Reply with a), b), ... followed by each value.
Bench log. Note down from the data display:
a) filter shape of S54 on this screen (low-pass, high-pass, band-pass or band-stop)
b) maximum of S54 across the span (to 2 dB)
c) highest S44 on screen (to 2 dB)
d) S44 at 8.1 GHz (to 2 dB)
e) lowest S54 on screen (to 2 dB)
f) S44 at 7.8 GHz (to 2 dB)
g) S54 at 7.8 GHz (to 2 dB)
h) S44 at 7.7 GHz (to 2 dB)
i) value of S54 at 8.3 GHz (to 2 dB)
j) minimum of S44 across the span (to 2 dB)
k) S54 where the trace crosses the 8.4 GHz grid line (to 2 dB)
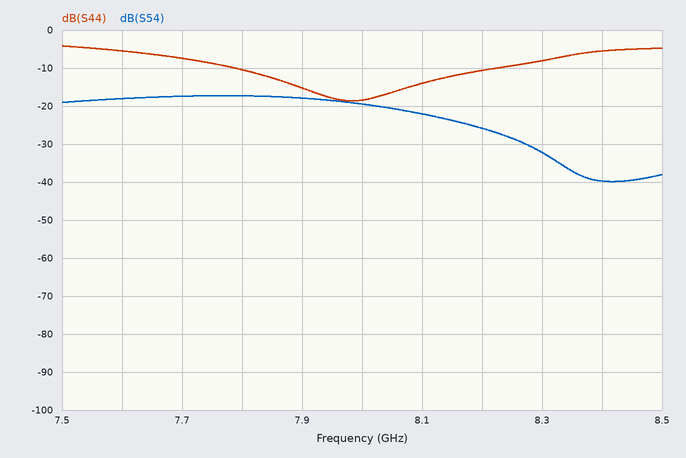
a) low-pass
b) -18 dB
c) -4 dB
d) -14 dB
e) -40 dB
f) -10 dB
g) -18 dB
h) -8 dB
i) -32 dB
j) -18 dB
k) -40 dB
